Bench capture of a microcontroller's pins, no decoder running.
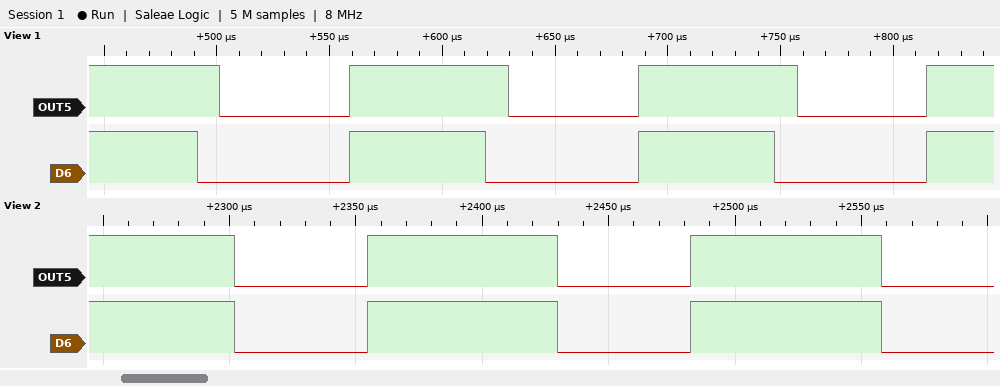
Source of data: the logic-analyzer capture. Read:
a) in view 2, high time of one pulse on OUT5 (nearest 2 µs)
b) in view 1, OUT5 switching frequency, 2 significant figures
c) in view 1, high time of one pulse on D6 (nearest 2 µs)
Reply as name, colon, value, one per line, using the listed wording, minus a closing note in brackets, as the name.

in view 2, high time of one pulse on OUT5: 76 µs
in view 1, OUT5 switching frequency, 2 significant figures: 7.8 kHz
in view 1, high time of one pulse on D6: 60 µs
